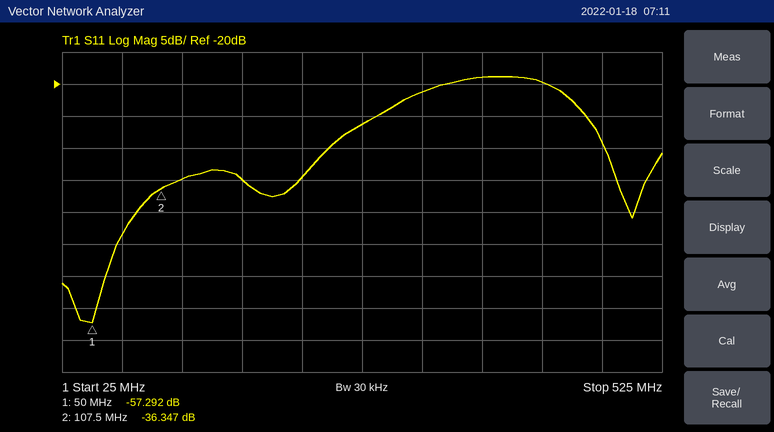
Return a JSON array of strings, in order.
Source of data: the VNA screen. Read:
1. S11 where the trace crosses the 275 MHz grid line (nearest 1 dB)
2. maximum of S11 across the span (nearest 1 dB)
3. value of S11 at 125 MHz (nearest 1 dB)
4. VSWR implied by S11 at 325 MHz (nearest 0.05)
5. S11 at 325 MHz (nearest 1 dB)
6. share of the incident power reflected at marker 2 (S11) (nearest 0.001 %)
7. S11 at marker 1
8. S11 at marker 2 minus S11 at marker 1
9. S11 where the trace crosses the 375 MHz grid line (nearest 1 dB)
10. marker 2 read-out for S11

["-26 dB", "-19 dB", "-35 dB", "1.20", "-21 dB", "0.023 %", "-57.292 dB", "20.945 dB", "-19 dB", "-36.347 dB"]
